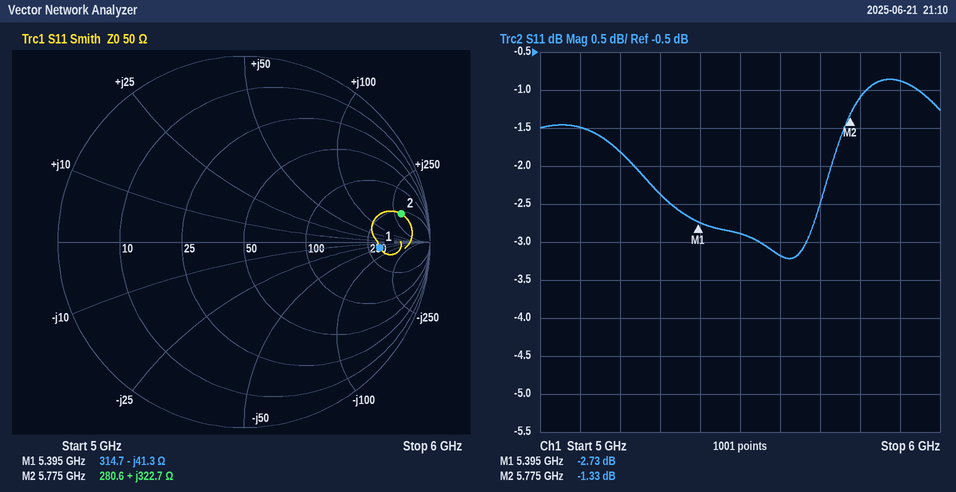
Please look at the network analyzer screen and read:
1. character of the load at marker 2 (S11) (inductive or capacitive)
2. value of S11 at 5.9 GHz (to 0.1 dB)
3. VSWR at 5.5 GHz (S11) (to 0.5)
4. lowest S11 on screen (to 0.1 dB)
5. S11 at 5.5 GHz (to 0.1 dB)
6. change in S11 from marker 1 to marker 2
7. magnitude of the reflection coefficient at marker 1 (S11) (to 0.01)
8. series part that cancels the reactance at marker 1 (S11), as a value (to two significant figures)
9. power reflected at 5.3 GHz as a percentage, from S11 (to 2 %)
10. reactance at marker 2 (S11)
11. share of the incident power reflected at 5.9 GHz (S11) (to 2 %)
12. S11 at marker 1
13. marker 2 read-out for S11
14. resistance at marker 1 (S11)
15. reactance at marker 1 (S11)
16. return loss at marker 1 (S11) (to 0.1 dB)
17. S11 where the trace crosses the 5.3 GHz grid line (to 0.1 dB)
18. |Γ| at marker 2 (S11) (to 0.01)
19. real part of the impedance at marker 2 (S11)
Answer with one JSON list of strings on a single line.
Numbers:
["inductive", "-0.9 dB", "6.0", "-3.2 dB", "-2.9 dB", "1.40 dB", "0.73", "1.2 nH", "58 %", "+322.7 Ω", "82 %", "-2.73 dB", "-1.33 dB", "314.7 Ω", "-41.3 Ω", "2.7 dB", "-2.4 dB", "0.86", "280.6 Ω"]
